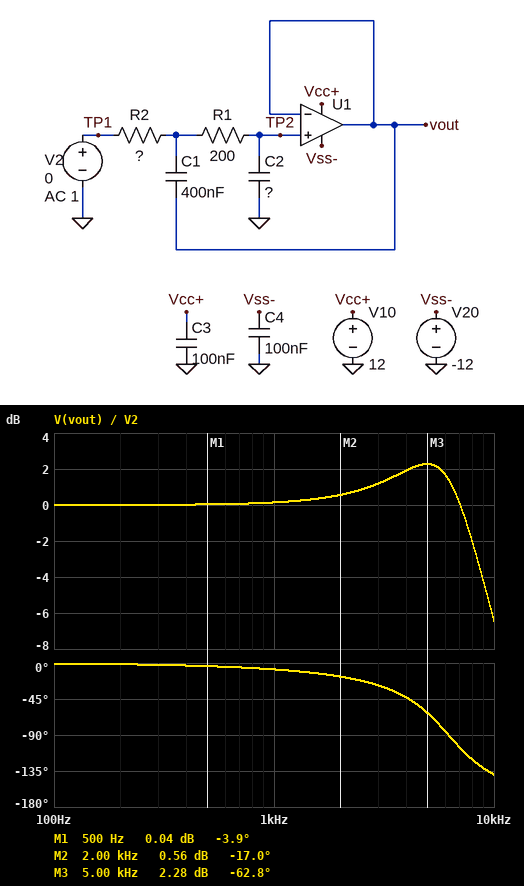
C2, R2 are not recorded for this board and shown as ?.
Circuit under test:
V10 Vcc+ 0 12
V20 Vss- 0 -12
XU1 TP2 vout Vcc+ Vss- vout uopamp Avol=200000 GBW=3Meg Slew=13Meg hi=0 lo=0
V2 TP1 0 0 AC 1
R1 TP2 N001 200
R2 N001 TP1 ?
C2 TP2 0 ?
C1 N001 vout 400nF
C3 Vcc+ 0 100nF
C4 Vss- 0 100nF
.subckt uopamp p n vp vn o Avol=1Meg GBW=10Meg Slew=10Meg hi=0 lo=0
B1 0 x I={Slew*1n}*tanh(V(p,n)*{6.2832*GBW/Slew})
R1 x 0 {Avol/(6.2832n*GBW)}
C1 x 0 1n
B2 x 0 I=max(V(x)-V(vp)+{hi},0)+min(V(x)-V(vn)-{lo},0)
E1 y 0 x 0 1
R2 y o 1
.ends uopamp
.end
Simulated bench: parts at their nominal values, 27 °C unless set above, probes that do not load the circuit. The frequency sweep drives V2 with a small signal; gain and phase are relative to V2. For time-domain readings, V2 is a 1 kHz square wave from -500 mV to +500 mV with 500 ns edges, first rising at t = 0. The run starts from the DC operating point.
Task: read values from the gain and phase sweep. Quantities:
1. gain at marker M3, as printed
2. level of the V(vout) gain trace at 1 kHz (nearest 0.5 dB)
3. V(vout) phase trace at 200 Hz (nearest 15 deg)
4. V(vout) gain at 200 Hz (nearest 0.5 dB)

2.28 dB
0 dB
0 deg
0 dB
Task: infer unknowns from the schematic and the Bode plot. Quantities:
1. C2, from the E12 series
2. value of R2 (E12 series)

68 nF
120 Ω
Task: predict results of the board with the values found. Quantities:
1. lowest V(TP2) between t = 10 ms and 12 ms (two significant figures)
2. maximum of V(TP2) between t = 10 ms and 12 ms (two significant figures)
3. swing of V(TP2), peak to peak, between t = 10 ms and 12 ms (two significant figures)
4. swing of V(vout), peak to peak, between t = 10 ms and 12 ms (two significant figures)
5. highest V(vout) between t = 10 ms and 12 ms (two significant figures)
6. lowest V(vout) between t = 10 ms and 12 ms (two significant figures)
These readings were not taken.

-730 mV
730 mV
1.5 V
1.5 V
730 mV
-730 mV
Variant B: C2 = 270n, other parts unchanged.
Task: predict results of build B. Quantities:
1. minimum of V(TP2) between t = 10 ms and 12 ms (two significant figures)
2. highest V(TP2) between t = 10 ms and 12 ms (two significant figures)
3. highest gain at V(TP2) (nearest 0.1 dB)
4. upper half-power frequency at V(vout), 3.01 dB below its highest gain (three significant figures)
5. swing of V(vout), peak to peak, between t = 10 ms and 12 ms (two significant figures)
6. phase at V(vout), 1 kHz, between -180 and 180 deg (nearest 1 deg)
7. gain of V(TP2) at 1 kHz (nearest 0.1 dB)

-510 mV
510 mV
0 dB
2.53 kHz
1.0 V
-31 deg
-0.4 dB
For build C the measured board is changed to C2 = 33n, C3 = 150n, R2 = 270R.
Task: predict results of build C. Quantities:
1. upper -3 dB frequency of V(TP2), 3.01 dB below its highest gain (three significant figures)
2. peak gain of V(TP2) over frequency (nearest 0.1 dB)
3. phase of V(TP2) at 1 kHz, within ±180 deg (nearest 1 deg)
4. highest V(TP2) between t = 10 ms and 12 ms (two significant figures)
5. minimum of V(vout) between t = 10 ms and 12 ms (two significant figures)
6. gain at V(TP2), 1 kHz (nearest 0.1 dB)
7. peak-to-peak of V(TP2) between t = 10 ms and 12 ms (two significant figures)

6.99 kHz
5.1 dB
-6 deg
890 mV
-890 mV
0.2 dB
1.8 V
